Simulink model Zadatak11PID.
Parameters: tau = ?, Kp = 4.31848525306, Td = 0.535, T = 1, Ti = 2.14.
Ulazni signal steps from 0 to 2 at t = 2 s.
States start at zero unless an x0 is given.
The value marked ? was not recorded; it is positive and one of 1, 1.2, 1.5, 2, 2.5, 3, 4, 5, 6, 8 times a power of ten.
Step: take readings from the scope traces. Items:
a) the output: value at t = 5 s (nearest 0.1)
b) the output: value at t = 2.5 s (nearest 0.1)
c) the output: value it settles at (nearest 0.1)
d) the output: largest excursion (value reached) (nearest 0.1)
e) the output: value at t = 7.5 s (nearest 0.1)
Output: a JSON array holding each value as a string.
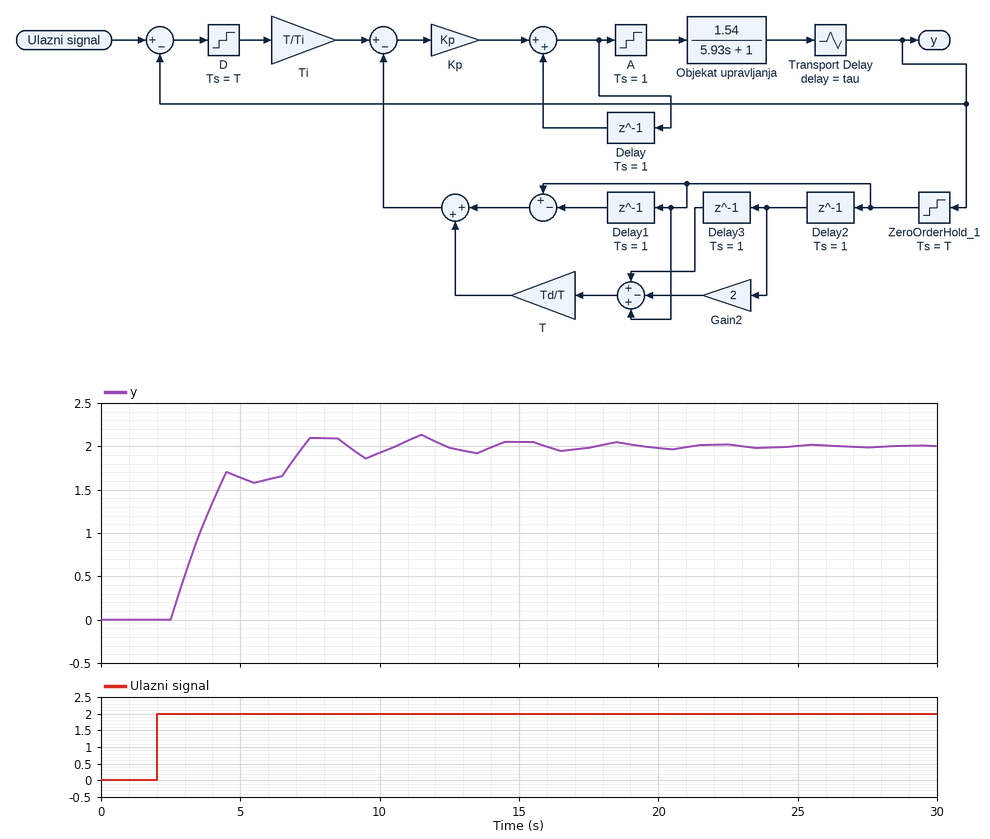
["1.6", "0.0", "2.0", "2.1", "2.1"]
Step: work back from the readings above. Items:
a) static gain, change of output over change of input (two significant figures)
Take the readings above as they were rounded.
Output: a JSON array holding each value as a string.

["1.0"]
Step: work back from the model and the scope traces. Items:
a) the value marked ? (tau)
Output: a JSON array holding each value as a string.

["0.5"]
